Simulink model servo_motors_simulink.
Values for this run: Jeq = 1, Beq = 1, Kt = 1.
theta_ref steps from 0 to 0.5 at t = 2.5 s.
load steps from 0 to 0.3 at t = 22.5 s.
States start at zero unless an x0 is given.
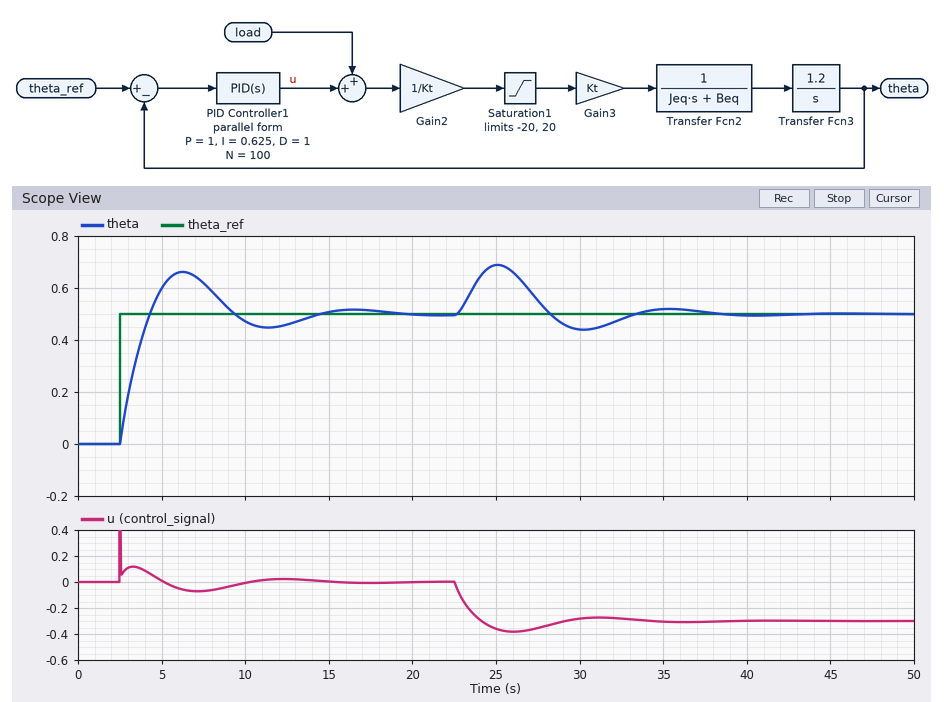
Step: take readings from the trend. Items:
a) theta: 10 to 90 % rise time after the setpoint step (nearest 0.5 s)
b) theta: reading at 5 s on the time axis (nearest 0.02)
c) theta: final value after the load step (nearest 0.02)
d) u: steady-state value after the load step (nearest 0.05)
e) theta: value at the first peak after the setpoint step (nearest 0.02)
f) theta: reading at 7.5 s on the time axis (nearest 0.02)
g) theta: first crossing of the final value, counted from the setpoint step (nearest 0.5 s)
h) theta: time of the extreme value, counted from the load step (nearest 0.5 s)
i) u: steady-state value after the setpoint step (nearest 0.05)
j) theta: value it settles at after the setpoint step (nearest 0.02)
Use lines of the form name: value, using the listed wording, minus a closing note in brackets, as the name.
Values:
theta: 10 to 90 % rise time after the setpoint step: 1.5 s
theta: reading at 5 s on the time axis: 0.60
theta: final value after the load step: 0.50
u: steady-state value after the load step: -0.30
theta: value at the first peak after the setpoint step: 0.66
theta: reading at 7.5 s on the time axis: 0.62
theta: first crossing of the final value, counted from the setpoint step: 2.0 s
theta: time of the extreme value, counted from the load step: 2.5 s
u: steady-state value after the setpoint step: 0.00
theta: value it settles at after the setpoint step: 0.50
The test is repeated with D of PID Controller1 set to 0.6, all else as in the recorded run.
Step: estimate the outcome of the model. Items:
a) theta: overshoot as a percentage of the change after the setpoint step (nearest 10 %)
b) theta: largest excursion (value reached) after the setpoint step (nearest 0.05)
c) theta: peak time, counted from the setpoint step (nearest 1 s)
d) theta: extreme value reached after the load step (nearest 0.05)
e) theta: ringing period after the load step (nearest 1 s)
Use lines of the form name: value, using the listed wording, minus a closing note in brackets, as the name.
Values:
theta: overshoot as a percentage of the change after the setpoint step: 40 %
theta: largest excursion (value reached) after the setpoint step: 0.70
theta: peak time, counted from the setpoint step: 3 s
theta: extreme value reached after the load step: 0.70
theta: ringing period after the load step: 9 s
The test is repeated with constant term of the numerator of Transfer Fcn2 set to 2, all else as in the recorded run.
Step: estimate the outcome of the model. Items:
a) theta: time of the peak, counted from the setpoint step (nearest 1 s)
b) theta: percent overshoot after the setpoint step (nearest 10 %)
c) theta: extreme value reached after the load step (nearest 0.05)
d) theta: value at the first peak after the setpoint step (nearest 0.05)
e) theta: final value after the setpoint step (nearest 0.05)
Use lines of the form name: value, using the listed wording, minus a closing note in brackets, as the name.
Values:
theta: time of the peak, counted from the setpoint step: 3 s
theta: percent overshoot after the setpoint step: 20 %
theta: extreme value reached after the load step: 0.70
theta: value at the first peak after the setpoint step: 0.60
theta: final value after the setpoint step: 0.50
